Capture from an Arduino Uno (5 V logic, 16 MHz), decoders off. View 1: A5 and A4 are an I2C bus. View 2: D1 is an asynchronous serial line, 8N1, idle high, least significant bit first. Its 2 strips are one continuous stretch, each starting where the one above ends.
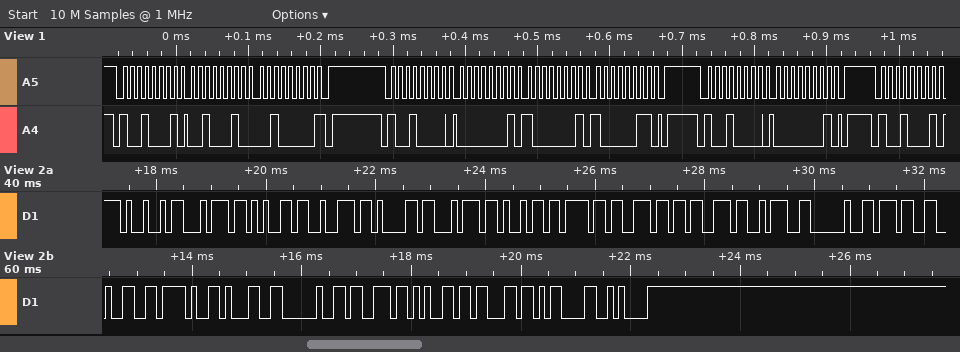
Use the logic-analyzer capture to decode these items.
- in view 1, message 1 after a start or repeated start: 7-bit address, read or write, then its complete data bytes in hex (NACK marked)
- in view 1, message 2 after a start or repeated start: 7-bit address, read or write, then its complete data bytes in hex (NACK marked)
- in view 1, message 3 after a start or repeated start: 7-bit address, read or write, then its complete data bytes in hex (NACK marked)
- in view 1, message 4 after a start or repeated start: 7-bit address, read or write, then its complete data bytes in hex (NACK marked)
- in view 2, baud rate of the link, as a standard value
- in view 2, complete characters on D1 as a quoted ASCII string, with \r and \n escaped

0x48 read: 22 20 NACK
0x48 write: 01 81 83
0x48 write: 01
0x48 read
9600 baud
"Iterations: 72/1 sec\r\n"
